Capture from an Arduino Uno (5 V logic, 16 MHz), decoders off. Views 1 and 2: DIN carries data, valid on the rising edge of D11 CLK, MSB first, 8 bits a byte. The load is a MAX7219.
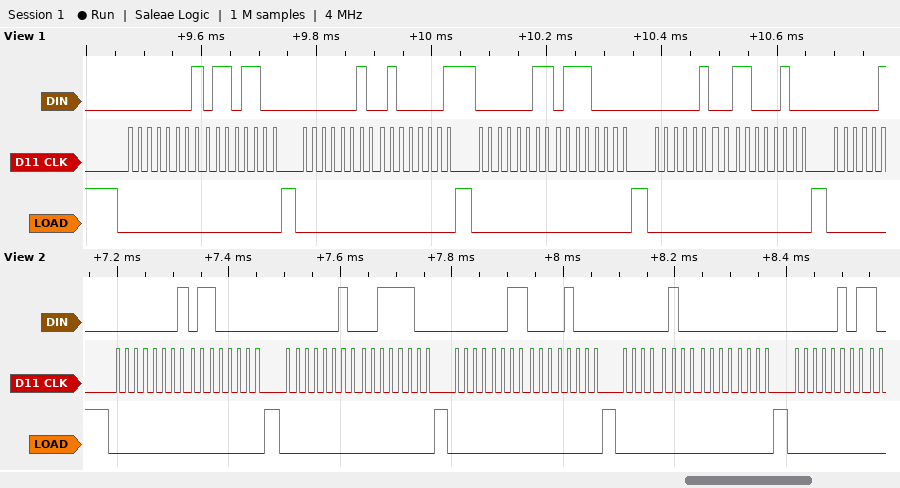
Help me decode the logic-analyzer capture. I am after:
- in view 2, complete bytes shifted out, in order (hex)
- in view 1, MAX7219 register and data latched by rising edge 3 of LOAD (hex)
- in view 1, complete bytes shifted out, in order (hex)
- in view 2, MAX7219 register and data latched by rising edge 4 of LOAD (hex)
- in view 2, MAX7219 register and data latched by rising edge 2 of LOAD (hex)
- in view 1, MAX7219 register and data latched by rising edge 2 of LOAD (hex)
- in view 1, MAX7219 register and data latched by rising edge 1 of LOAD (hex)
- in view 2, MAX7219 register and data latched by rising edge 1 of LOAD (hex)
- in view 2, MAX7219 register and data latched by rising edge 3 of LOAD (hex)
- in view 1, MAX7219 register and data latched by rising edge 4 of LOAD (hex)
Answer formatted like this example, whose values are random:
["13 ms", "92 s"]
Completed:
["01 60 02 3C 03 08 04 00 05", "register 0x3, data 0x70", "0x01 0x6C 0x02 0x41 0x03 0x70 0x04 0xC4", "register 0x4, data 0x00", "register 0x2, data 0x3C", "register 0x2, data 0x41", "register 0x1, data 0x6C", "register 0x1, data 0x60", "register 0x3, data 0x08", "register 0x4, data 0xC4"]
